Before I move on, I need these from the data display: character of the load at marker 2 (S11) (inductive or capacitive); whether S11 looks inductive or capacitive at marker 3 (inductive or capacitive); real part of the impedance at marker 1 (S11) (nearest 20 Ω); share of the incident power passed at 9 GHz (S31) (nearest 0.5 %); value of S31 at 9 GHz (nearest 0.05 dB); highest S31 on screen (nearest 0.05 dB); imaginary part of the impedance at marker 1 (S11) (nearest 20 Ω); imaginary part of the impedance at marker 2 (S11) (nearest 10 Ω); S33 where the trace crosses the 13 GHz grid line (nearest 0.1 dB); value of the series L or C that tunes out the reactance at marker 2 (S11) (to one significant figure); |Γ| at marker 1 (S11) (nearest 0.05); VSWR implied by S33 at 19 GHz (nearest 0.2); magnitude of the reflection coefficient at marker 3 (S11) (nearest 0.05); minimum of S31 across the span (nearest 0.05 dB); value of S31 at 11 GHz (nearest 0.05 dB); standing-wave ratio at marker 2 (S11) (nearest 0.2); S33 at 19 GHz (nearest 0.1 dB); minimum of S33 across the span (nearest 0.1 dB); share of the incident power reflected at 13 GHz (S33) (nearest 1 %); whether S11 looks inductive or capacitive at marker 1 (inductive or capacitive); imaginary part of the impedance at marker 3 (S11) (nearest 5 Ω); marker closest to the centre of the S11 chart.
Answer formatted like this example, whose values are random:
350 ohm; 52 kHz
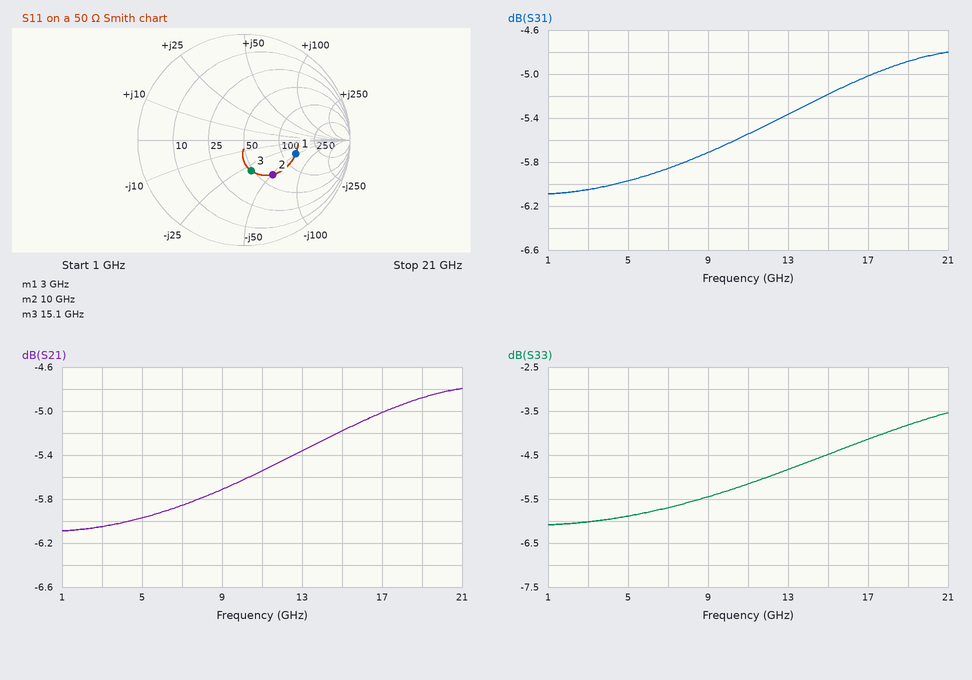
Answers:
capacitive; capacitive; 140 Ω; 27.0 %; -5.70 dB; -4.80 dB; -40 Ω; -50 Ω; -4.8 dB; 800 pH; 0.50; 4.6; 0.30; -6.10 dB; -5.55 dB; 2.4; -3.8 dB; -6.1 dB; 33 %; capacitive; -30 Ω; marker 3
